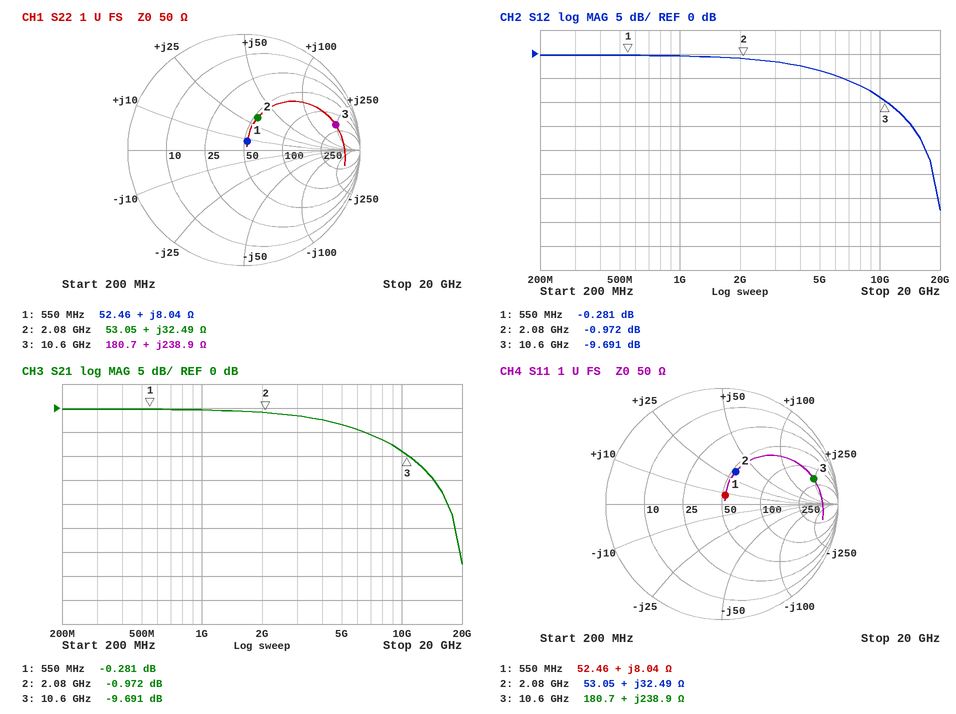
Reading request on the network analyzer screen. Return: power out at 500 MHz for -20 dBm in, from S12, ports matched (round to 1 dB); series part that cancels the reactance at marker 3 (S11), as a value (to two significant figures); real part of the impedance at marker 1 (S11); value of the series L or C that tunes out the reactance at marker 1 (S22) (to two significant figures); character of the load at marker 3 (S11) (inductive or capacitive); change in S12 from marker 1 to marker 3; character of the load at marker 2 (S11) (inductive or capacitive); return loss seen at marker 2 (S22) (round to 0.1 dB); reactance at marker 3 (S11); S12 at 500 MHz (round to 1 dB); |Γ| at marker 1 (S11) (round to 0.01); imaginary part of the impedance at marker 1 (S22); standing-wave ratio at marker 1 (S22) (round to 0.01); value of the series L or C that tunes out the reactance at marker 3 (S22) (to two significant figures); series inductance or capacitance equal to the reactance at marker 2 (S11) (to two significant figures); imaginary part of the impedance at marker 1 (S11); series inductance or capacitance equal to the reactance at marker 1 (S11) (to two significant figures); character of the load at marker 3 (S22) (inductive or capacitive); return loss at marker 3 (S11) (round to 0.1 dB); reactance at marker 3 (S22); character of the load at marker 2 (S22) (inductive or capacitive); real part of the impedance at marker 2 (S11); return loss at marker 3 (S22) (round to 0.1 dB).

-20 dBm
63 fF
52.46 Ω
36 pF
inductive
-9.410 dB
inductive
10.4 dB
+238.9 Ω
0 dB
0.08
+8.04 Ω
1.18
63 fF
2.5 nH
+8.04 Ω
2.3 nH
inductive
1.7 dB
+238.9 Ω
inductive
53.05 Ω
1.7 dB
